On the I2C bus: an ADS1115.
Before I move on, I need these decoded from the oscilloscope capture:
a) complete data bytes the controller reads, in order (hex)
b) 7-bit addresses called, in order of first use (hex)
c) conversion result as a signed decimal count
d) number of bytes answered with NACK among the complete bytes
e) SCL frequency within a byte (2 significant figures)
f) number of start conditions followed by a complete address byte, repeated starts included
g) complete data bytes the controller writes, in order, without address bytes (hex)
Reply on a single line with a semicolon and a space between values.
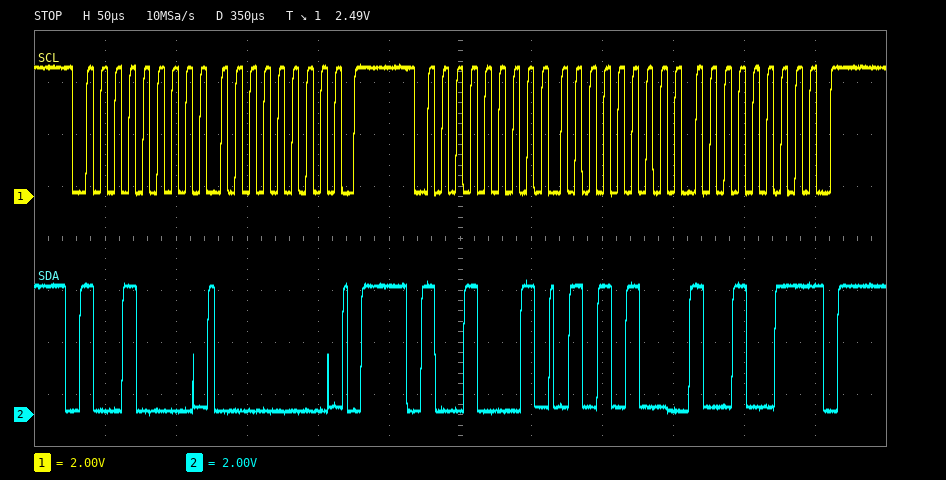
54 93; 0x48; 21651; 1; 100 kHz; 2; 00
